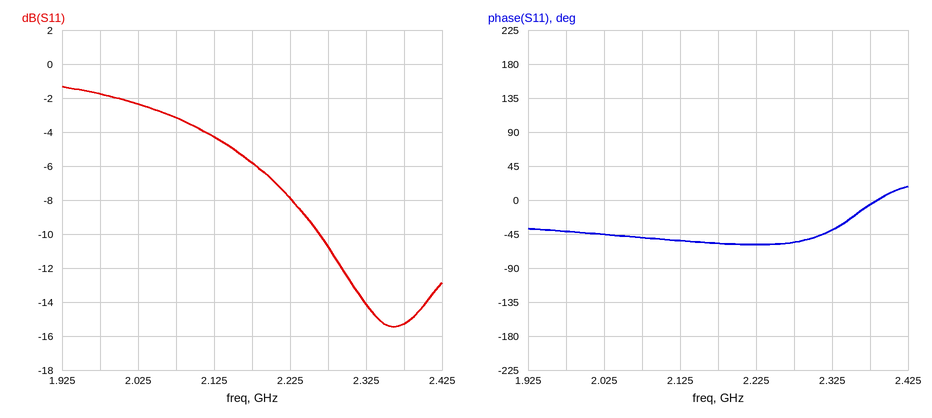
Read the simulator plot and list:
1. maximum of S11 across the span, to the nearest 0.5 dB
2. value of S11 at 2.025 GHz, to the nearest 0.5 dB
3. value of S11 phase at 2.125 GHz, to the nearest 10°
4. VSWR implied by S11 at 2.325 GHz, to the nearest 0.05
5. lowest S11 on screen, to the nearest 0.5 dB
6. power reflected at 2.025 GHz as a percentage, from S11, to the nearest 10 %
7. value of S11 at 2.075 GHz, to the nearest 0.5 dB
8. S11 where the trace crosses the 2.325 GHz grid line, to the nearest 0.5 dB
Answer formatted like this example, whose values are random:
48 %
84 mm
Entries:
-1.5 dB
-2.5 dB
-50°
1.50
-15.5 dB
60 %
-3.0 dB
-14.0 dB
